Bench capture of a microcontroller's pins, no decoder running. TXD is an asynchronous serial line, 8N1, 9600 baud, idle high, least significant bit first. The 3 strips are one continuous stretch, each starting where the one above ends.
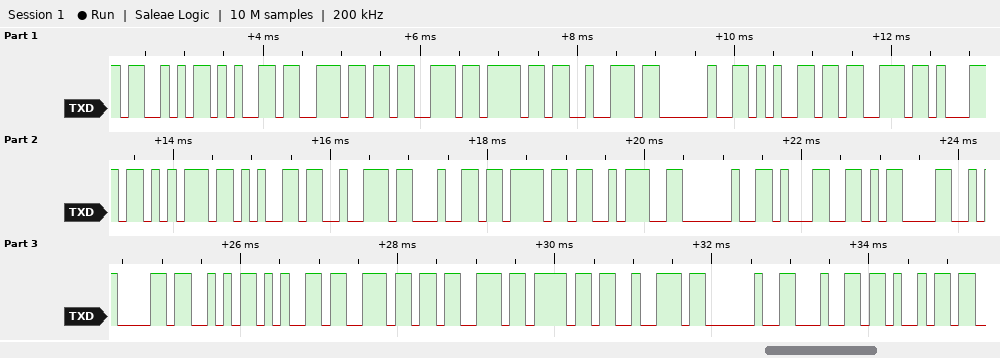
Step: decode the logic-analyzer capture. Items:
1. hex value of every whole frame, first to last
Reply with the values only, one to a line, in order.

53 65 6E 73 6F 72 20 65 73 71 75 65 72 64 6F 3A 20 31 0D 0A 53 65 6E 73 6F 72 20 64 69
